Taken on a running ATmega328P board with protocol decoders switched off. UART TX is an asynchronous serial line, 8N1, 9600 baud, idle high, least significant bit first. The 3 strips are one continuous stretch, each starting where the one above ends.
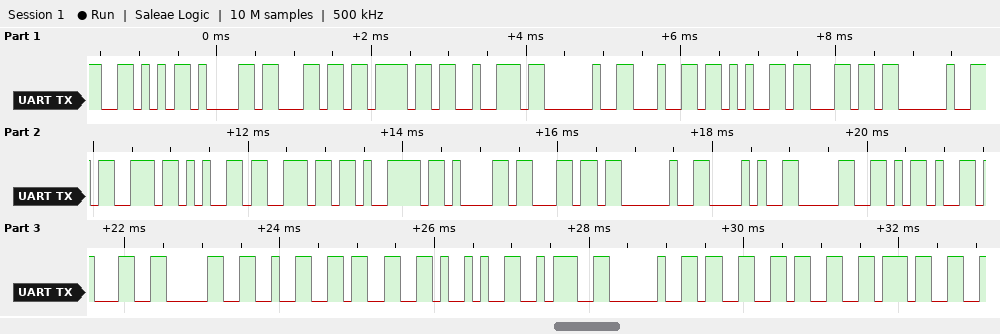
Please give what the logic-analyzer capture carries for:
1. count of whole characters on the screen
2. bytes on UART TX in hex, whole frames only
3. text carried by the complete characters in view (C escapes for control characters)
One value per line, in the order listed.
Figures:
30
56 61 6C 6F 72 20 64 65 6C 20 73 65 6E 79 61 6C 20 28 30 2D 31 30 32 33 29 3A 20 33 33 37
"Valor del senyal (0-1023): 337"
